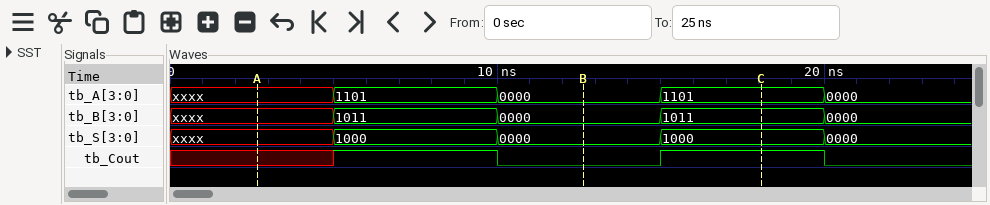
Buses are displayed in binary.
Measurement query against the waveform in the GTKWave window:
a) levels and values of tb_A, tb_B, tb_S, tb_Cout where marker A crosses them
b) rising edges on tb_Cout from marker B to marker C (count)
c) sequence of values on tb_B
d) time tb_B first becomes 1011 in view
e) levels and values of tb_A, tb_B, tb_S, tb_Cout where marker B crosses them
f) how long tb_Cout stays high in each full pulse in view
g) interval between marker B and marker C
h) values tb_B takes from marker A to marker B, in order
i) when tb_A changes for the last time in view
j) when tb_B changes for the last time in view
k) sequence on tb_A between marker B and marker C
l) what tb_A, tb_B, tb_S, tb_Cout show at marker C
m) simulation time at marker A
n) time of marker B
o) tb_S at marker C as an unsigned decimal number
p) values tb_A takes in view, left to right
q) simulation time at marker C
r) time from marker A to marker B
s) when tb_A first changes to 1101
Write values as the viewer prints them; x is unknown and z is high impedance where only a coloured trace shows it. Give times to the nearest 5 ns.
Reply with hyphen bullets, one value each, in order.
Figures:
- tb_A=xxxx, tb_B=xxxx, tb_S=xxxx, tb_Cout=x
- 1
- xxxx, 1011, 0000, 1011, 0000
- 5 ns
- tb_A=0000, tb_B=0000, tb_S=0000, tb_Cout=0
- 5 ns
- 5 ns
- xxxx, 1011, 0000
- 20 ns
- 20 ns
- 0000, 1101
- tb_A=1101, tb_B=1011, tb_S=1000, tb_Cout=1
- 5 ns
- 15 ns
- 8
- xxxx, 1101, 0000, 1101, 0000
- 20 ns
- 10 ns
- 5 ns
